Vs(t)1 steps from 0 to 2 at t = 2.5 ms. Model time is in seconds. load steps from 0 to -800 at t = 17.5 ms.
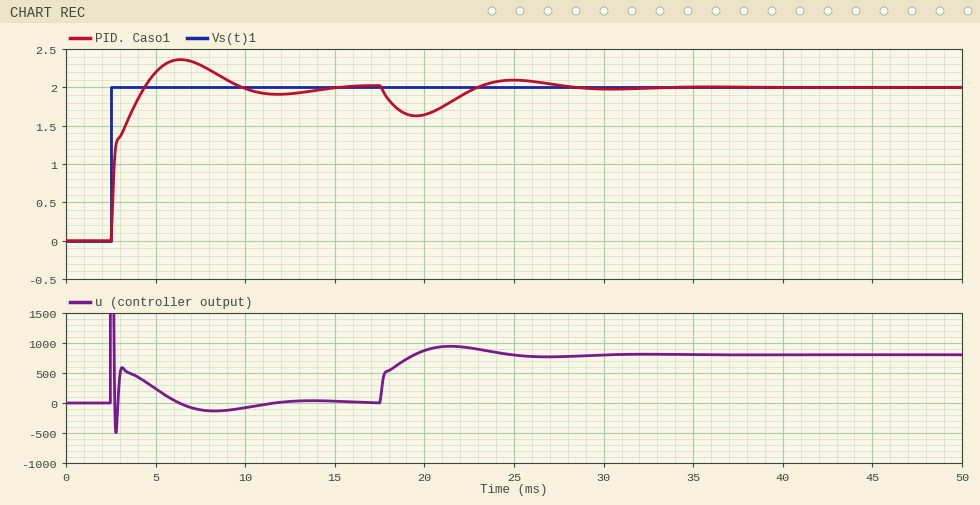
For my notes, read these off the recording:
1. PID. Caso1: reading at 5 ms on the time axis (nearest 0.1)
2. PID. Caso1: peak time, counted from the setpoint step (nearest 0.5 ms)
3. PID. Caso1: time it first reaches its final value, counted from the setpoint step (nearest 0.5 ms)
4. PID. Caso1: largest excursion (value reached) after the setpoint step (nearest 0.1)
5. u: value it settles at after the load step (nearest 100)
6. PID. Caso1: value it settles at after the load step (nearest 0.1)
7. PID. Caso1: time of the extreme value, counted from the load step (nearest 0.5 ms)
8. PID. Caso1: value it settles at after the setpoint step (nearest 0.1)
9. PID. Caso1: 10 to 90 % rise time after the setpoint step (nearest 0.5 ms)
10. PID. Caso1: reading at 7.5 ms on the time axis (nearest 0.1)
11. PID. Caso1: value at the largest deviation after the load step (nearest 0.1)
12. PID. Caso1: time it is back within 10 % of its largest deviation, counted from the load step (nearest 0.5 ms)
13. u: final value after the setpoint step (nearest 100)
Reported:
2.2
4.0 ms
2.0 ms
2.4
800
2.0
2.0 ms
2.0
1.5 ms
2.3
1.6
9.5 ms
0
